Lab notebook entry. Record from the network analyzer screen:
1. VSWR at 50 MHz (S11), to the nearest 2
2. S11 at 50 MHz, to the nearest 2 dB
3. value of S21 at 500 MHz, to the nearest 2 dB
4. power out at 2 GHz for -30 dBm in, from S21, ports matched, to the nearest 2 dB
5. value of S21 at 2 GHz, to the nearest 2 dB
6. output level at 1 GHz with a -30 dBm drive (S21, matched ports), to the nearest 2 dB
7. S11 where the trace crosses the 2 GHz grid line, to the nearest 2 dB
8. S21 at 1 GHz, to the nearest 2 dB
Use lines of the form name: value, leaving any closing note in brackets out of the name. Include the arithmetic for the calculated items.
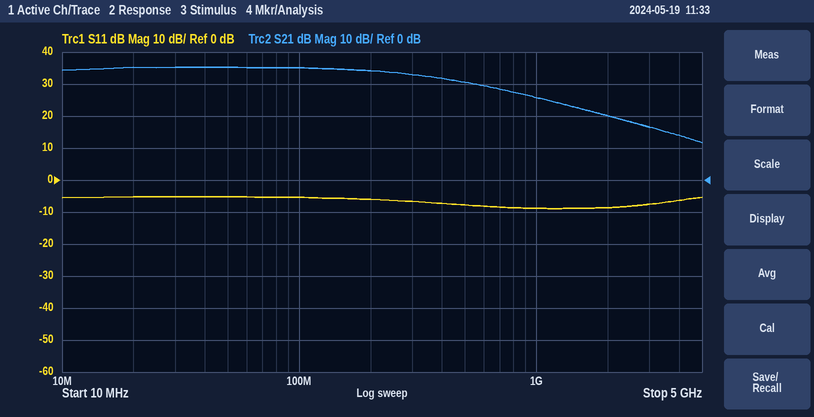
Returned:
VSWR at 50 MHz (S11), to the nearest 2: |Γ| = 10^(-6/20) = 0.5012; VSWR = (1 + 0.5012)/(1 − 0.5012) ≈ 3.01, so 4 to the nearest 2
S11 at 50 MHz, to the nearest 2 dB: -6 dB
value of S21 at 500 MHz, to the nearest 2 dB: 30 dB
power out at 2 GHz for -30 dBm in, from S21, ports matched, to the nearest 2 dB: -30 dBm + (20 dB) = -10 dBm
value of S21 at 2 GHz, to the nearest 2 dB: 20 dB
output level at 1 GHz with a -30 dBm drive (S21, matched ports), to the nearest 2 dB: -30 dBm + (26 dB) = -4 dBm
S11 where the trace crosses the 2 GHz grid line, to the nearest 2 dB: -8 dB
S21 at 1 GHz, to the nearest 2 dB: 26 dB
